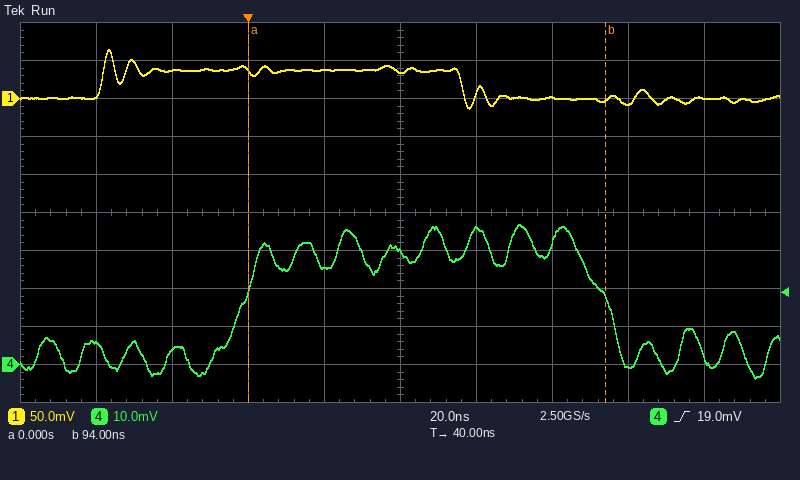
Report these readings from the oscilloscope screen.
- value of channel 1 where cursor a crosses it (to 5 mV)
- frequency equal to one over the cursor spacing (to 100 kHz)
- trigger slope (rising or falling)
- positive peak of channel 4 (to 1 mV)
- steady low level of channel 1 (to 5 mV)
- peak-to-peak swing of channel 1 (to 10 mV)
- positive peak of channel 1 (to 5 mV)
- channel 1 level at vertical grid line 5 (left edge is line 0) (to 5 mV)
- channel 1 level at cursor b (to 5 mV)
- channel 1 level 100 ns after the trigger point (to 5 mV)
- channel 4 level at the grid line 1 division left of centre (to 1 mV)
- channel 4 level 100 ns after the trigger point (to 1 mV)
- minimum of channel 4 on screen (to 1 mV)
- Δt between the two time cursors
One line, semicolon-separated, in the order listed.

35 mV; 10.6 MHz; rising; 37 mV; 0 mV; 80 mV; 65 mV; 35 mV; 0 mV; -5 mV; 26 mV; 0 mV; -4 mV; 94 ns
